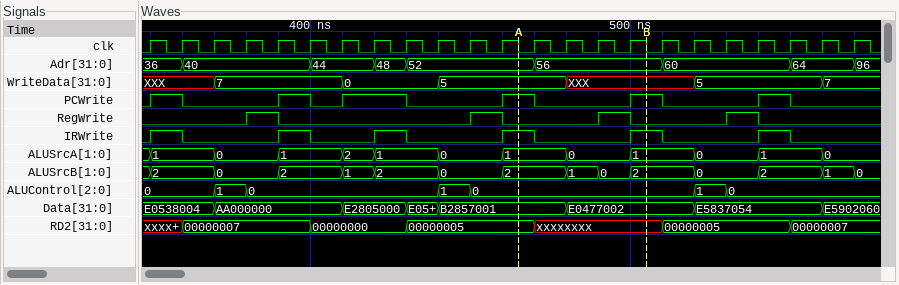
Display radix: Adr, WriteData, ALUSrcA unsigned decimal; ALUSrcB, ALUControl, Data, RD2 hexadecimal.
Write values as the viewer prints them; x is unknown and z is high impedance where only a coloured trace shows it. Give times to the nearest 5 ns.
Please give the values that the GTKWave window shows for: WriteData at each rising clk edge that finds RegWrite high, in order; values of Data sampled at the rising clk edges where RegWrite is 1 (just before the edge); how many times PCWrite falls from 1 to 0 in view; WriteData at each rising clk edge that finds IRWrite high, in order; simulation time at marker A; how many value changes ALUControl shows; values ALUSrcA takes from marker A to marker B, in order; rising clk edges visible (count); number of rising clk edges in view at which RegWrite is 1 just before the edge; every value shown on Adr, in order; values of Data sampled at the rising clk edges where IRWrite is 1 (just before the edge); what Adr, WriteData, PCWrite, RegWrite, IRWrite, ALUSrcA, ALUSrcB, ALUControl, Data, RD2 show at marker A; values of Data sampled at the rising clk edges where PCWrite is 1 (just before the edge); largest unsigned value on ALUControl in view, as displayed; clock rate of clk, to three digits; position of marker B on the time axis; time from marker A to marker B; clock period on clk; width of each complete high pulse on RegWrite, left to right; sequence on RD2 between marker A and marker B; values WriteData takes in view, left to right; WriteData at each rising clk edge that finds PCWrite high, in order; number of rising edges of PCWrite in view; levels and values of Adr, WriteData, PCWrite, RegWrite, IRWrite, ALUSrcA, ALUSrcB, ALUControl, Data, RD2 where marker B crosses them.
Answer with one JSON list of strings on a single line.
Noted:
["7, 5, XXX, 5", "AA000000, B2857001, E0477002, E5837054", "6", "XXX, 7, 0, 5, XXX, 5", "465 ns", "6", "1, 0, 1", "23", "4", "36, 40, 44, 48, 52, 56, 60, 64, 96", "E0538004, AA000000, E2805000, B2857001, E0477002, E5837054", "Adr=52, WriteData=5, PCWrite=1, RegWrite=0, IRWrite=1, ALUSrcA=1, ALUSrcB=2, ALUControl=0, Data=B2857001, RD2=00000005", "E0538004, AA000000, E2805000, E2805000, B2857001, E0477002, E5837054", "1", "100 MHz", "505 ns", "40 ns", "10 ns", "10 ns, 10 ns, 10 ns, 10 ns", "00000005, xxxxxxxx", "XXX, 7, 0, 5, XXX, 5, 7", "XXX, 7, 0, 0, 5, XXX, 5", "6", "Adr=56, WriteData=XXX, PCWrite=1, RegWrite=0, IRWrite=1, ALUSrcA=1, ALUSrcB=2, ALUControl=0, Data=E0477002, RD2=xxxxxxxx"]
